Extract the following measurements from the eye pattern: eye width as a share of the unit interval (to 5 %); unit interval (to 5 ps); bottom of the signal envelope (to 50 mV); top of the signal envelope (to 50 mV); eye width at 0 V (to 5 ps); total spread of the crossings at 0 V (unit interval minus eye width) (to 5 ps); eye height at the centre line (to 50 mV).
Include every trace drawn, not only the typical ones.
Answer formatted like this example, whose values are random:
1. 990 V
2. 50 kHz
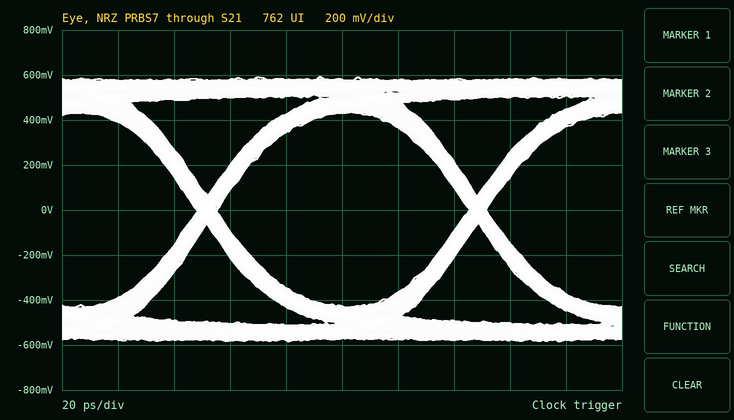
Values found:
1. 95 %
2. 95 ps
3. -600 mV
4. 600 mV
5. 90 ps
6. 5 ps
7. 850 mV
